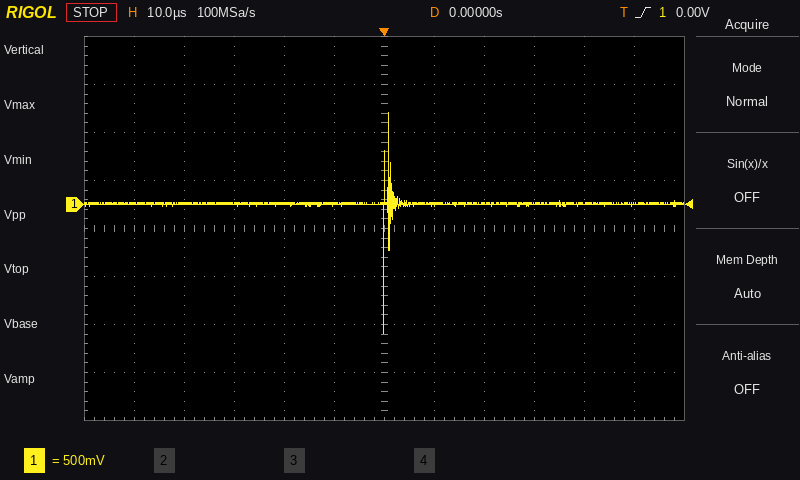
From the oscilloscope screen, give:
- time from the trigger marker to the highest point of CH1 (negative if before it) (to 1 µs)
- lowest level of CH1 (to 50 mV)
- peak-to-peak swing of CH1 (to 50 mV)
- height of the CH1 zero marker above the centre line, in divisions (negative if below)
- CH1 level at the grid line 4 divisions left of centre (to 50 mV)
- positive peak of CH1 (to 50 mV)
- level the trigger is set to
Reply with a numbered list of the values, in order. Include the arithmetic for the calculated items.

1. +1 µs
2. -1.35 V
3. 950 mV − (-1.35 V) = 2.30 V
4. +0.5 div
5. 0 mV
6. 950 mV
7. 0.00 V
